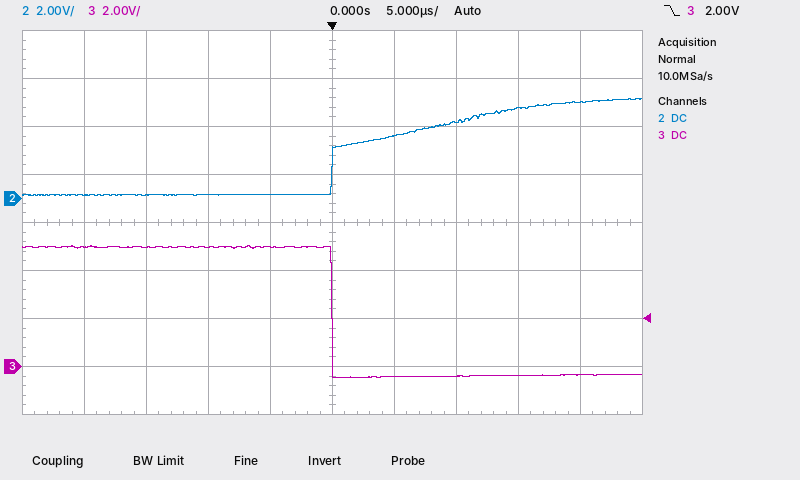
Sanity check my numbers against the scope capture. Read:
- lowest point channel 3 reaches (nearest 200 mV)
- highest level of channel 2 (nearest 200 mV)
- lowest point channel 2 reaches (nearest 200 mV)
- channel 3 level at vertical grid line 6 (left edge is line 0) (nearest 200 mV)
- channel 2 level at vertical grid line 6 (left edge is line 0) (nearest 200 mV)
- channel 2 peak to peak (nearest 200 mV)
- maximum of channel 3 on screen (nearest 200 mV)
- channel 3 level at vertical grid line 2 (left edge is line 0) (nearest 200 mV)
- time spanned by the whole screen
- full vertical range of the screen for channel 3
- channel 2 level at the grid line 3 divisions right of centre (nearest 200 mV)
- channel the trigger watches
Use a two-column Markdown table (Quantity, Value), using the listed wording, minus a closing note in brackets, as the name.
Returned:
| Quantity | Value |
|---|---|
| lowest point channel 3 reaches | -400 mV |
| highest level of channel 2 | 4.2 V |
| lowest point channel 2 reaches | 200 mV |
| channel 3 level at vertical grid line 6 (left edge is line 0) | -400 mV |
| channel 2 level at vertical grid line 6 (left edge is line 0) | 2.6 V |
| channel 2 peak to peak | 4.0 V |
| maximum of channel 3 on screen | 5.0 V |
| channel 3 level at vertical grid line 2 (left edge is line 0) | 5.0 V |
| time spanned by the whole screen | 50 µs |
| full vertical range of the screen for channel 3 | 16 V |
| channel 2 level at the grid line 3 divisions right of centre | 3.8 V |
| channel the trigger watches | channel 3 |
